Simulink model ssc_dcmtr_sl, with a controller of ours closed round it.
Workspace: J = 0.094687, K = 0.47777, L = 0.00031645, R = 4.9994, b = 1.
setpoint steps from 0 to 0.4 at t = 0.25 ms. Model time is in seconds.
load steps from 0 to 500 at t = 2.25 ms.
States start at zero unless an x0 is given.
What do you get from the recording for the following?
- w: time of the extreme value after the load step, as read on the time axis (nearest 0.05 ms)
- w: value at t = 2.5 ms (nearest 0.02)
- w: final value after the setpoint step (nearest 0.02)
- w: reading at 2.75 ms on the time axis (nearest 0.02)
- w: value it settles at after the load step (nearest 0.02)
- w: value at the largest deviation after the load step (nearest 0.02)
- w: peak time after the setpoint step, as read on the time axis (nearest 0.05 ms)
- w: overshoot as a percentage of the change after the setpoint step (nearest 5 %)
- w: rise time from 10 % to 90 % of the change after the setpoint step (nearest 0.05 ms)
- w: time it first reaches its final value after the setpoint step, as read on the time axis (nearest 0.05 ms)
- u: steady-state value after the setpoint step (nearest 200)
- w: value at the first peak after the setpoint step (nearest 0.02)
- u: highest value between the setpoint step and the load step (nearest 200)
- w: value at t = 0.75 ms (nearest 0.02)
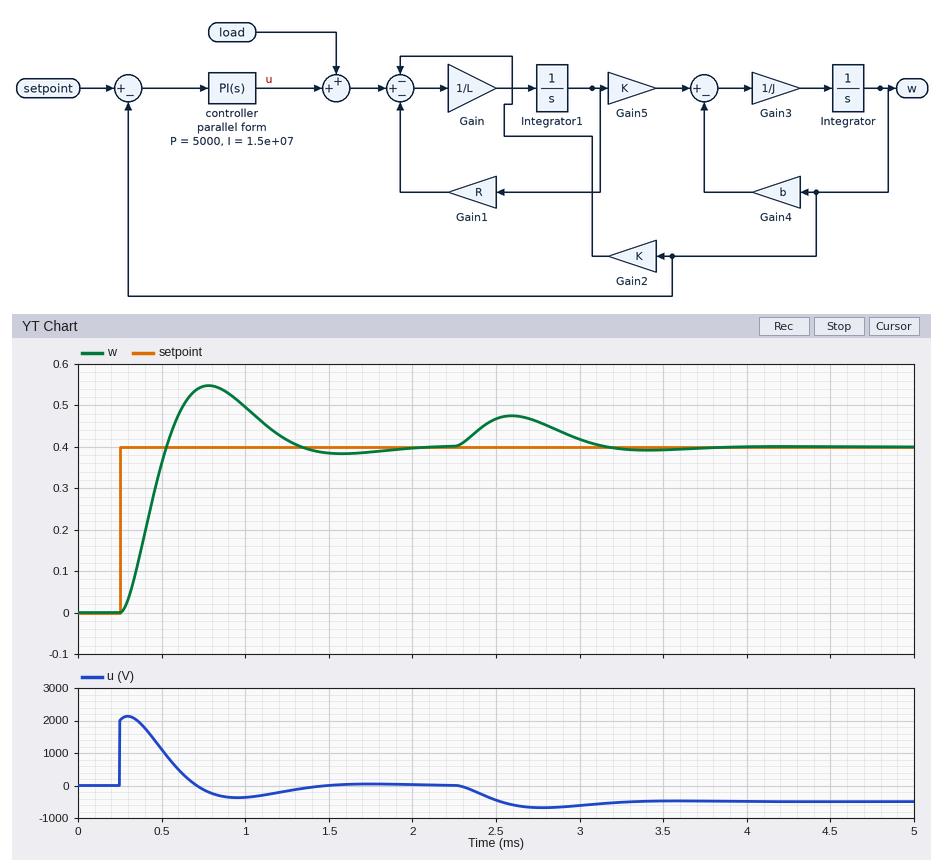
2.60 ms
0.46
0.40
0.46
0.40
0.48
0.80 ms
35 %
0.20 ms
0.55 ms
0
0.54
2200
0.54
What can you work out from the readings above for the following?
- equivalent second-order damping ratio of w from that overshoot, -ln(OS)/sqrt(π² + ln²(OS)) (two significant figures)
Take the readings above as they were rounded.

0.32
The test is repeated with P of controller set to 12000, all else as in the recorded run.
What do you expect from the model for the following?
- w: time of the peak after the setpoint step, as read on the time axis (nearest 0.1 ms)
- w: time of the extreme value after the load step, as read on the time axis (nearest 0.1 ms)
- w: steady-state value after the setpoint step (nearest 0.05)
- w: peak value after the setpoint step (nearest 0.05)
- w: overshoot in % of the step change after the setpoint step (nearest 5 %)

0.5 ms
2.5 ms
0.40
0.50
25 %
